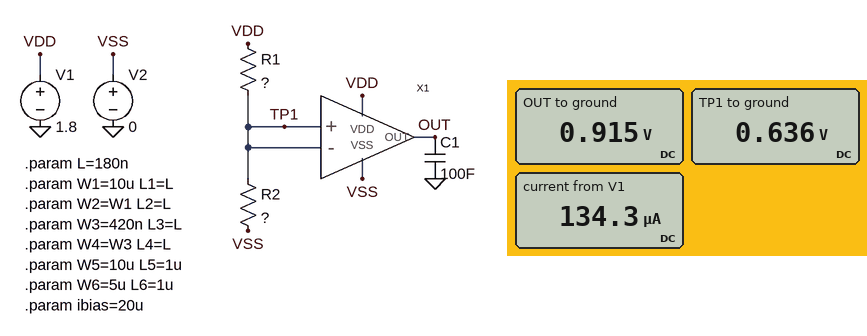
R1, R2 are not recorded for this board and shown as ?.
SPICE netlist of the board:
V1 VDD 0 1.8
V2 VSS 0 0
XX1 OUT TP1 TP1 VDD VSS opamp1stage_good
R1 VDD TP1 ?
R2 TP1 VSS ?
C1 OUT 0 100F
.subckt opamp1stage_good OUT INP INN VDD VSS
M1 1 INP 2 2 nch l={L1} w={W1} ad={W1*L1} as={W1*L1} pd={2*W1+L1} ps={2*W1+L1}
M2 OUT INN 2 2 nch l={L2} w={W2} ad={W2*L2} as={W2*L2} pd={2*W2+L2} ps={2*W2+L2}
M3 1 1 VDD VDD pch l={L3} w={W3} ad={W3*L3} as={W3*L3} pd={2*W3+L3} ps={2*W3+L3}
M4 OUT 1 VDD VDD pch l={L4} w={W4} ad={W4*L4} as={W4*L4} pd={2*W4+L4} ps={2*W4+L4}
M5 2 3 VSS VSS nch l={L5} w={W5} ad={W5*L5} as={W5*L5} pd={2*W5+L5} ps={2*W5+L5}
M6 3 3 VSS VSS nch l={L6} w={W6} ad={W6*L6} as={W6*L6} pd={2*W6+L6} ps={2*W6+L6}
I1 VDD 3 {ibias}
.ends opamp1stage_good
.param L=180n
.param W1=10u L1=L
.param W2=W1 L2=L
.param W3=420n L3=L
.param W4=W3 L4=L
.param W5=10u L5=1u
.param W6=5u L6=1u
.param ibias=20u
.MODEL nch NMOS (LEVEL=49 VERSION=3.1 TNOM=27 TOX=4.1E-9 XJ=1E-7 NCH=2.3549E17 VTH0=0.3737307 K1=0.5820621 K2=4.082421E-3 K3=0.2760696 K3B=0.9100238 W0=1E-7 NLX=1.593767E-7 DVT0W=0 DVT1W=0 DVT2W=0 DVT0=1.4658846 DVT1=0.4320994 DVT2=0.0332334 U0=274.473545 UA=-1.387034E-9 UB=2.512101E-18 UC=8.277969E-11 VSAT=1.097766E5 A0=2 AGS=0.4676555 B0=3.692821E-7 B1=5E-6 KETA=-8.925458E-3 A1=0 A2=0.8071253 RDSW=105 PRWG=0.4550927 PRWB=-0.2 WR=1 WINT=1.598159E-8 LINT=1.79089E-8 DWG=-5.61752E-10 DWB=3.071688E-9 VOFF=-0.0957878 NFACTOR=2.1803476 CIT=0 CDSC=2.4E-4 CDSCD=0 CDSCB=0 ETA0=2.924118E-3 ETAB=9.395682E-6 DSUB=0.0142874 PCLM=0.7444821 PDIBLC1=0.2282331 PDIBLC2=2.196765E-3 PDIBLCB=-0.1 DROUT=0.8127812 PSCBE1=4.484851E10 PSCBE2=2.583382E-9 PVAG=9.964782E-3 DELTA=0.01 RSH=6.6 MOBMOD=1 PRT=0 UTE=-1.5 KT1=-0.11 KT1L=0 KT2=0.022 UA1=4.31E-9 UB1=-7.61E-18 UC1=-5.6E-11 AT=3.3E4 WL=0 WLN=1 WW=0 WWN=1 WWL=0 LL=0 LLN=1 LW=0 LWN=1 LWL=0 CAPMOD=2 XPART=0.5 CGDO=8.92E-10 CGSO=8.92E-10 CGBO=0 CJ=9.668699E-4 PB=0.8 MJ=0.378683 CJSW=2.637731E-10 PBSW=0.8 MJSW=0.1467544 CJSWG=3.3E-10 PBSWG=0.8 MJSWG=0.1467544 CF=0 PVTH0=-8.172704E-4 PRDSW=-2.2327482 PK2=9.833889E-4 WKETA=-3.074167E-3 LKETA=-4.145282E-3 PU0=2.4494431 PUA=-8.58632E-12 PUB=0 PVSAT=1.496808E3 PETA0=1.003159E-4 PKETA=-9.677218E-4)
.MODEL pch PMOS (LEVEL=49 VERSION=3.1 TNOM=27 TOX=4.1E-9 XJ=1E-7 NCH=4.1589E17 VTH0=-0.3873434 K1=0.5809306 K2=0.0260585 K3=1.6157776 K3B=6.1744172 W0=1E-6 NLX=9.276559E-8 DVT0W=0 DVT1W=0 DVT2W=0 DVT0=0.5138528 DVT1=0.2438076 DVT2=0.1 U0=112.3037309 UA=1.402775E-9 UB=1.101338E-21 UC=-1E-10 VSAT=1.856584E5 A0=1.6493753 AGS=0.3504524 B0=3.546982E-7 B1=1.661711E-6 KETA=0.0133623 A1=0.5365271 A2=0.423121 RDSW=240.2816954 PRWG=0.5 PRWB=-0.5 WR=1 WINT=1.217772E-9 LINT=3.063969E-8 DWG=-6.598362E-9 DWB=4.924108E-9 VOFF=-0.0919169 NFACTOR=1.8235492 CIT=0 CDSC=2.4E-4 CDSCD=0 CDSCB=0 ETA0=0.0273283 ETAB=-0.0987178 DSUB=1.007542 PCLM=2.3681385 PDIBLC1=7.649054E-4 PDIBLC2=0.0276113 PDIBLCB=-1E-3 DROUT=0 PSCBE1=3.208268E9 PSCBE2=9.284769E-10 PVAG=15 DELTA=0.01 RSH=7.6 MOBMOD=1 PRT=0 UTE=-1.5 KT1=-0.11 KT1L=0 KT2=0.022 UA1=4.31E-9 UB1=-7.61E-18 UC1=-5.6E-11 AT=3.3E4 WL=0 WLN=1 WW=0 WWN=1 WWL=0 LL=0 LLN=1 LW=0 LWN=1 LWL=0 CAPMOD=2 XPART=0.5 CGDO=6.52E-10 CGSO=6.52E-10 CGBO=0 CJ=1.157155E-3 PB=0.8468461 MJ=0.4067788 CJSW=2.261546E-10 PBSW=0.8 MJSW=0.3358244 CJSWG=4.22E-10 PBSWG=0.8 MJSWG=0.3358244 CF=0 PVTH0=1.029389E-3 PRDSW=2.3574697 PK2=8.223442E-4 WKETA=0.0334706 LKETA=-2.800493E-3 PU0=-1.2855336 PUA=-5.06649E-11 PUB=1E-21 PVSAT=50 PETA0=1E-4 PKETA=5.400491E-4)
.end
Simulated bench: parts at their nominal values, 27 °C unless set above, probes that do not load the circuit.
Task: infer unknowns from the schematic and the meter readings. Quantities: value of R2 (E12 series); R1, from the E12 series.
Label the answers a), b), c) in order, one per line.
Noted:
a) 8.2 kΩ
b) 15 kΩ
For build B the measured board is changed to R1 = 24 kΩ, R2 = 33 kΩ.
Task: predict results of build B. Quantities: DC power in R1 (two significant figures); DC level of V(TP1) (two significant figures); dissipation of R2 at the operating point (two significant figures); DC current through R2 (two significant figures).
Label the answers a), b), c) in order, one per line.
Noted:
a) 24 µW
b) 1.0 V
c) 33 µW
d) 32 µA
